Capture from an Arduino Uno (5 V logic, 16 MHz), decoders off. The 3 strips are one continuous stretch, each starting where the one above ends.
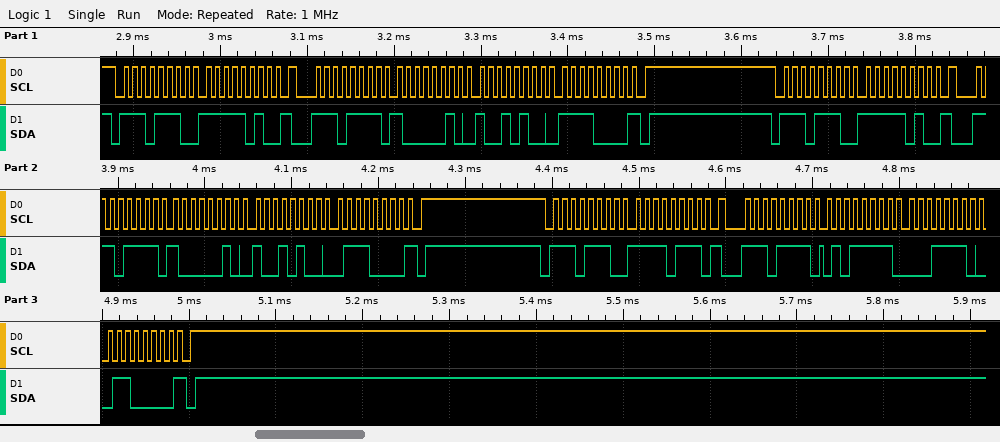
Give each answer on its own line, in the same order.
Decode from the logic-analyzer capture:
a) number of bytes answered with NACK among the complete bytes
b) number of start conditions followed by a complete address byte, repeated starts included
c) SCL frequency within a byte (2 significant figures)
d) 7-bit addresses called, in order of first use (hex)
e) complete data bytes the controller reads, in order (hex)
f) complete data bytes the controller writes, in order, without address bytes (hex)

3
6
100 kHz
0x77
82 94 F0 82 94 70 5F 1E 60
FA FA F7
